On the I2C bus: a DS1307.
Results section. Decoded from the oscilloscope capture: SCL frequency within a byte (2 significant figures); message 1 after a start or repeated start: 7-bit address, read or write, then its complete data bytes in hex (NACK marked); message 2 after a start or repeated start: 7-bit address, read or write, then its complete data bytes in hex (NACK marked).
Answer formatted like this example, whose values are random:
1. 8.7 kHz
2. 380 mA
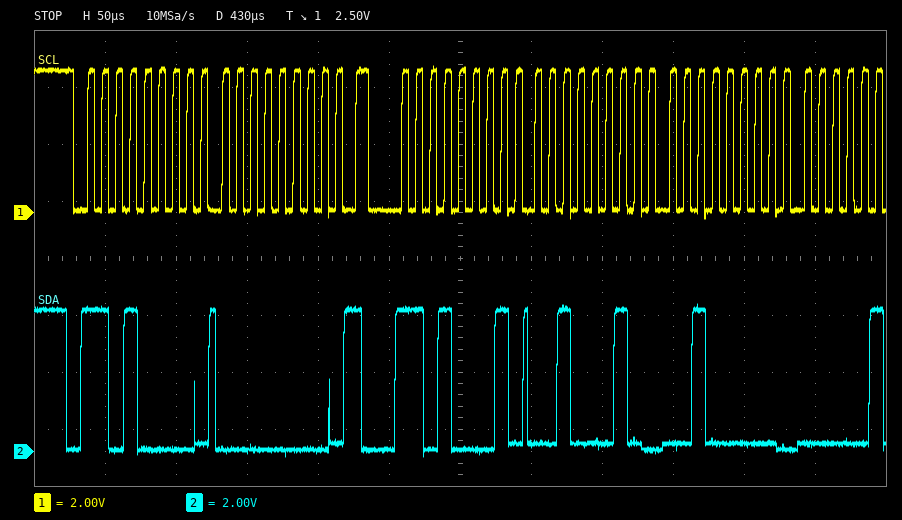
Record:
1. 100 kHz
2. 0x68 write: 00
3. 0x68 read: 22 20
